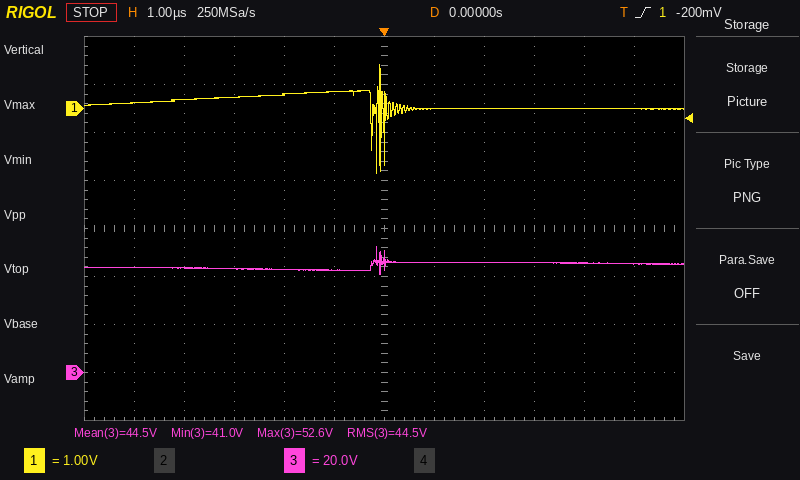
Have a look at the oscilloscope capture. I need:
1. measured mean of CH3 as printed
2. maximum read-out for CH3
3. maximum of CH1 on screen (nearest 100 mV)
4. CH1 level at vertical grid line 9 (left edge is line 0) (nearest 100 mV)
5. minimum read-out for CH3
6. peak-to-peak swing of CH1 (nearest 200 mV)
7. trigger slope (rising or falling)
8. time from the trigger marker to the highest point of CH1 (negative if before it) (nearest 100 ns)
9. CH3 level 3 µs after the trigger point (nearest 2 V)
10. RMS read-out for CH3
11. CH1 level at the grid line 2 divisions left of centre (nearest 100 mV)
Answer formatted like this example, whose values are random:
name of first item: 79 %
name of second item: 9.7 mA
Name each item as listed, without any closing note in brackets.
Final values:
measured mean of CH3 as printed: 44.5 V
maximum read-out for CH3: 52.6 V
maximum of CH1 on screen: 900 mV
CH1 level at vertical grid line 9 (left edge is line 0): 0.0 V
minimum read-out for CH3: 41.0 V
peak-to-peak swing of CH1: 2.2 V
trigger slope: rising
time from the trigger marker to the highest point of CH1 (negative if before it): -100 ns
CH3 level 3 µs after the trigger point: 46 V
RMS read-out for CH3: 44.5 V
CH1 level at the grid line 2 divisions left of centre: 300 mV
